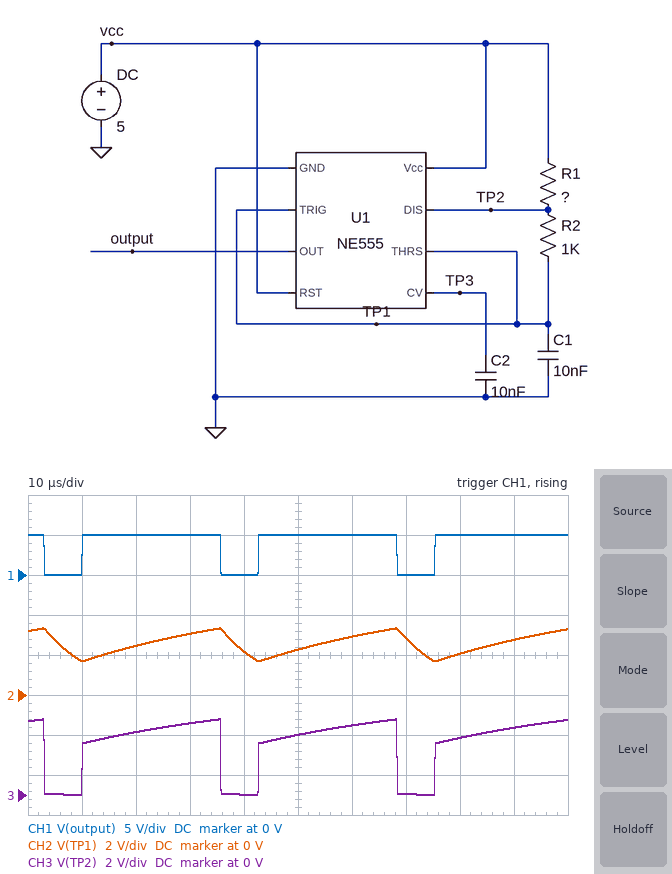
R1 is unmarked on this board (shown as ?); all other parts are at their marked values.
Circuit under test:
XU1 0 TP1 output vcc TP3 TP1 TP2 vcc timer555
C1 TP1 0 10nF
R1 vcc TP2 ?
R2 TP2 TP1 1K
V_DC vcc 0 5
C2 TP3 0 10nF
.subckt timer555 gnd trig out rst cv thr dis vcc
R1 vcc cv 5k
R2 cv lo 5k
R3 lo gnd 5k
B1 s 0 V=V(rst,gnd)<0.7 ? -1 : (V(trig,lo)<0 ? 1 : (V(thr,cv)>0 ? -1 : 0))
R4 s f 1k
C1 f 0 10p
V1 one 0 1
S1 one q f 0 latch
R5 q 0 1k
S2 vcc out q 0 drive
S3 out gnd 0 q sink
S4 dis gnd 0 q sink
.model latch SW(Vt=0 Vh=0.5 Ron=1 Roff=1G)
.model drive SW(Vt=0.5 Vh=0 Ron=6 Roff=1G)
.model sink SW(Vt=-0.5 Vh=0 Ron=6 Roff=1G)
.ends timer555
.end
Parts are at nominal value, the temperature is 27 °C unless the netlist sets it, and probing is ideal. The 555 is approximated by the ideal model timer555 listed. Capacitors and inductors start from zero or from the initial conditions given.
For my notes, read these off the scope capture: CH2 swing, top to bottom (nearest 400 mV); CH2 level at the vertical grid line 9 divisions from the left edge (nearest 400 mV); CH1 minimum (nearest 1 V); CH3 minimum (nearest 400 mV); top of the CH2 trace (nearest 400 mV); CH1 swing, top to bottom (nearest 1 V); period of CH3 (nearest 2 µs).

1.6 V
2.8 V
0 V
0 V
3.2 V
5 V
32 µs
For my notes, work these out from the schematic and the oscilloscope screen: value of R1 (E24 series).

2.7 kΩ
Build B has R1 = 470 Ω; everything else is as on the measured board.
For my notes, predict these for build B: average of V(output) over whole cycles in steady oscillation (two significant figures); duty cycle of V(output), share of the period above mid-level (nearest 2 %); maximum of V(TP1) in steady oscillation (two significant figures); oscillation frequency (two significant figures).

2.9 V
58 %
3.3 V
58 kHz
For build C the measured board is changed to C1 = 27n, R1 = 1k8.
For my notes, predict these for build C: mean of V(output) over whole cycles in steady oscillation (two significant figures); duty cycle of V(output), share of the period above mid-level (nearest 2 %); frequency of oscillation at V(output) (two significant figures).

3.7 V
74 %
14 kHz
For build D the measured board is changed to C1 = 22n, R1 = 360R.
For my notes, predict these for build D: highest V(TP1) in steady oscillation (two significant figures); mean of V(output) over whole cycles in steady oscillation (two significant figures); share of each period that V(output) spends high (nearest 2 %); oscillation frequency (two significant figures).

3.3 V
2.8 V
56 %
27 kHz
